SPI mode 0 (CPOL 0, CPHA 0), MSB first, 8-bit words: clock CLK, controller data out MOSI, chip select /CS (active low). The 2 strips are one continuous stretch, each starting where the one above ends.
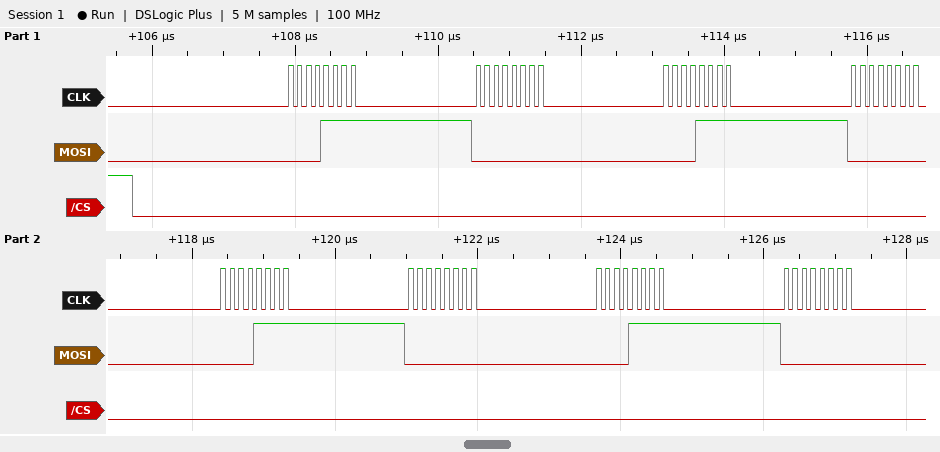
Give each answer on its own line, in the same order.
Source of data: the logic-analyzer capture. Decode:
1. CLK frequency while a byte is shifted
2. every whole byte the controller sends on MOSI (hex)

8 MHz
0F 00 0F 00 0F 00 0F 00
